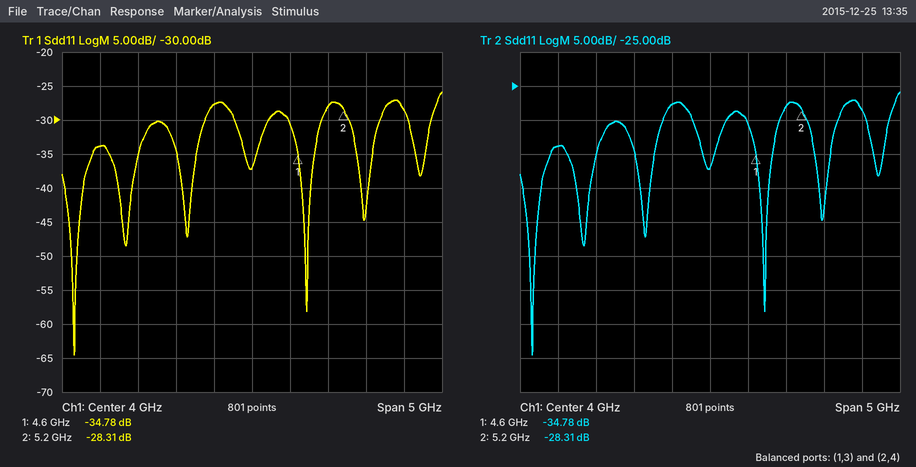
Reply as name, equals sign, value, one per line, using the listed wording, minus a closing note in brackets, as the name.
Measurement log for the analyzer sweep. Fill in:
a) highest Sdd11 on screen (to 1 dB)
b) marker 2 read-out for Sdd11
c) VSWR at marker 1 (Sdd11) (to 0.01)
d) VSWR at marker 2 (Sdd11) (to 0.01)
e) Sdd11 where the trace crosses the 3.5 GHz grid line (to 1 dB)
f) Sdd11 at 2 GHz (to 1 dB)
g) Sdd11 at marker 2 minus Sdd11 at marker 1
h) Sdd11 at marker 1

highest Sdd11 on screen = -26 dB
marker 2 read-out for Sdd11 = -28.31 dB
VSWR at marker 1 (Sdd11) = 1.04
VSWR at marker 2 (Sdd11) = 1.08
Sdd11 where the trace crosses the 3.5 GHz grid line = -28 dB
Sdd11 at 2 GHz = -34 dB
Sdd11 at marker 2 minus Sdd11 at marker 1 = 6.47 dB
Sdd11 at marker 1 = -34.78 dB
